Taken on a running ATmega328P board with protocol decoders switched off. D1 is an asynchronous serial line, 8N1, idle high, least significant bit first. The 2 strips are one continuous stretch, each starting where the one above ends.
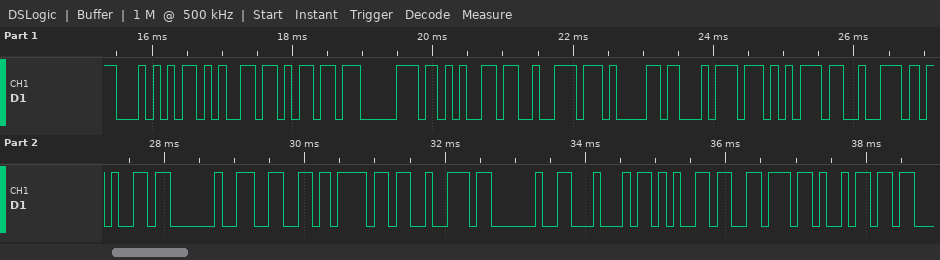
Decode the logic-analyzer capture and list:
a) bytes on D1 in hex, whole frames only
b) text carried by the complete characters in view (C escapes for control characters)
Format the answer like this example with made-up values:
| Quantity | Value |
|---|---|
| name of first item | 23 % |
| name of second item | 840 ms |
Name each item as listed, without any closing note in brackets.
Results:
| Quantity | Value |
|---|---|
| bytes on D1 in hex, whole frames only | 54 65 6D 70 65 72 61 74 75 72 65 20 66 6F 72 20 44 65 76 69 |
| text carried by the complete characters in view | "Temperature for Devi" |
